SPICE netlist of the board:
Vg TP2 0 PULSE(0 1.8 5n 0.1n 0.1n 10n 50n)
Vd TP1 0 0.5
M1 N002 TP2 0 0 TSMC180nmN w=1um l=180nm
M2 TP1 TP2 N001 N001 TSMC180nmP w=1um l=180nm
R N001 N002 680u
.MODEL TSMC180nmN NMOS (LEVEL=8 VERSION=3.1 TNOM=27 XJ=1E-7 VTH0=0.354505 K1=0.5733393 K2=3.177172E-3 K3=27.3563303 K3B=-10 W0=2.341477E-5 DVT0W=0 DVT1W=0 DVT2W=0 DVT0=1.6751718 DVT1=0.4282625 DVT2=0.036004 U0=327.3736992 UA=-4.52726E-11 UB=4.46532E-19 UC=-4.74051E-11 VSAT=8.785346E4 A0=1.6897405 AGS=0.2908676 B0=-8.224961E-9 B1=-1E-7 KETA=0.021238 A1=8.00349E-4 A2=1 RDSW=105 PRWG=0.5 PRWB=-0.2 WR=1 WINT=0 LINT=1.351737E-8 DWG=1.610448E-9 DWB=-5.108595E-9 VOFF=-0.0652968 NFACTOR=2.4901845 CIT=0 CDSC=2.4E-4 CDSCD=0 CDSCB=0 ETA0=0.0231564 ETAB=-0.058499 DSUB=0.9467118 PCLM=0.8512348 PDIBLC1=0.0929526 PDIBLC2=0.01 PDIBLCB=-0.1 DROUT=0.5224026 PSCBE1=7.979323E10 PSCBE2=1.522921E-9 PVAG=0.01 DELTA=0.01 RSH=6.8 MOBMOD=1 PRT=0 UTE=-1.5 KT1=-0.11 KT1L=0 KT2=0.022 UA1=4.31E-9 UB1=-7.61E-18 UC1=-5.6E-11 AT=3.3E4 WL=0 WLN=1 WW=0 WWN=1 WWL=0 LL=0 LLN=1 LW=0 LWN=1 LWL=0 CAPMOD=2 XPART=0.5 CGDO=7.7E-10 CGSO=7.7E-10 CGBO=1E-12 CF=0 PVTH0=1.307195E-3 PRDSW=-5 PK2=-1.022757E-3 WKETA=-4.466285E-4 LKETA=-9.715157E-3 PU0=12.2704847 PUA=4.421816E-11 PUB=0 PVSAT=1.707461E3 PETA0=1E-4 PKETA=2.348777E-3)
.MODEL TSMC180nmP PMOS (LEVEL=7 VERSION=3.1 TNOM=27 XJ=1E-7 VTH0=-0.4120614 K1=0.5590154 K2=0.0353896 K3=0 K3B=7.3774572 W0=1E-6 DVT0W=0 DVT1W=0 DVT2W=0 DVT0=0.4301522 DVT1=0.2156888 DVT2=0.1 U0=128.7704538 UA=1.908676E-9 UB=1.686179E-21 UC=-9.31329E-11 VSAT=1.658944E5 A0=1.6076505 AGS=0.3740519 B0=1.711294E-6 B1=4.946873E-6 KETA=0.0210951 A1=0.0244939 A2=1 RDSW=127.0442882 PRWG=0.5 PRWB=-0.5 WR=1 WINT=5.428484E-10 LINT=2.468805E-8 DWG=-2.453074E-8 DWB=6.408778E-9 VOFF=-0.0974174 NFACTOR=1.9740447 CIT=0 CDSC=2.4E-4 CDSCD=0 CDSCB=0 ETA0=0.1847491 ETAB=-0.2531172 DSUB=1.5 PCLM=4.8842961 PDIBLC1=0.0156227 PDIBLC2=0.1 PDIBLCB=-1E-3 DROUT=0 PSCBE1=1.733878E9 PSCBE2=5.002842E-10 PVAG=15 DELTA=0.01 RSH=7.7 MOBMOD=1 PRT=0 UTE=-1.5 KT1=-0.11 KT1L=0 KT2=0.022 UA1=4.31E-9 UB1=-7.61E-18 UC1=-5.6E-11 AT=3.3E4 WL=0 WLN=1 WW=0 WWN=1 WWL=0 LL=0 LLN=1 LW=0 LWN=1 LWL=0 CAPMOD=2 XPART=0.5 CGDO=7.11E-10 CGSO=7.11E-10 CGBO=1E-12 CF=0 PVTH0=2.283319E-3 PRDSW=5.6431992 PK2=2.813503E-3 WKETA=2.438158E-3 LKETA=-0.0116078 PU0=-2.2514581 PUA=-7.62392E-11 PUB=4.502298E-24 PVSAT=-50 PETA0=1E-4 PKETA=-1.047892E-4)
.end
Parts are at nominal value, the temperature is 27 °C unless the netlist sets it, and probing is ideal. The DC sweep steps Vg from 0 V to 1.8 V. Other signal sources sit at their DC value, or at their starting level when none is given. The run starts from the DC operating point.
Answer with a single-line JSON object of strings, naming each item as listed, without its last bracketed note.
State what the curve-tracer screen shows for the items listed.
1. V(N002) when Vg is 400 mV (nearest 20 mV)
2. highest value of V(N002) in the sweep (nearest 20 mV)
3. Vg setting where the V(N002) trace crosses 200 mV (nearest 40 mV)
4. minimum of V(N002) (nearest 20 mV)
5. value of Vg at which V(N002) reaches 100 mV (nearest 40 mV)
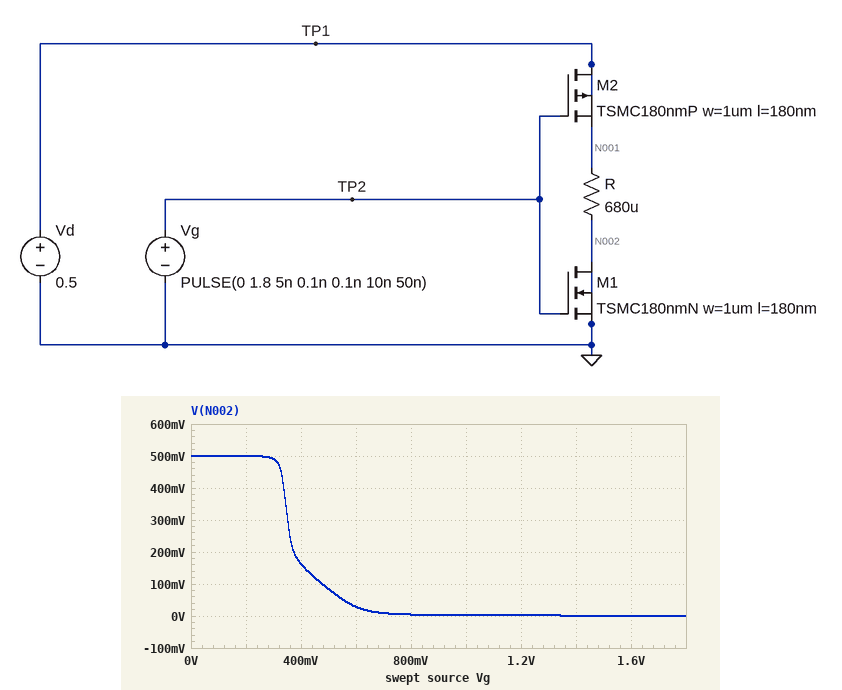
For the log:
{"V(N002) when Vg is 400 mV": "160 mV", "highest value of V(N002) in the sweep": "500 mV", "Vg setting where the V(N002) trace crosses 200 mV": "360 mV", "minimum of V(N002)": "0 V", "value of Vg at which V(N002) reaches 100 mV": "480 mV"}
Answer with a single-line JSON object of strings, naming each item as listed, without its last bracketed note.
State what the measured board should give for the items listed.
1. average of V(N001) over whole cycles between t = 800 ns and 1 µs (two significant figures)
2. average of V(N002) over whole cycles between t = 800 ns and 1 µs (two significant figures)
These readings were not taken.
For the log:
{"average of V(N001) over whole cycles between t = 800 ns and 1 µs": "390 mV", "average of V(N002) over whole cycles between t = 800 ns and 1 µs": "390 mV"}
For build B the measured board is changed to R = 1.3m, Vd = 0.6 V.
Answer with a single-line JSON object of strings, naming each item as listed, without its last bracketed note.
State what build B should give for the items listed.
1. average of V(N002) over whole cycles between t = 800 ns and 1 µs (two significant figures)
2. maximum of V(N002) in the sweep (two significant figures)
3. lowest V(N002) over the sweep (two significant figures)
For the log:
{"average of V(N002) over whole cycles between t = 800 ns and 1 µs": "480 mV", "maximum of V(N002) in the sweep": "600 mV", "lowest V(N002) over the sweep": "23 mV"}
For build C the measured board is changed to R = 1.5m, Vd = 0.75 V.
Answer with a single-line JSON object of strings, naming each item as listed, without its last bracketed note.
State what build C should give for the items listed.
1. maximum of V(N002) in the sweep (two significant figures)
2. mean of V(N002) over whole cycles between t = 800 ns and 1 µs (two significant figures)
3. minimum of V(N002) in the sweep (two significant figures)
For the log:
{"maximum of V(N002) in the sweep": "750 mV", "mean of V(N002) over whole cycles between t = 800 ns and 1 µs": "620 mV", "minimum of V(N002) in the sweep": "130 mV"}
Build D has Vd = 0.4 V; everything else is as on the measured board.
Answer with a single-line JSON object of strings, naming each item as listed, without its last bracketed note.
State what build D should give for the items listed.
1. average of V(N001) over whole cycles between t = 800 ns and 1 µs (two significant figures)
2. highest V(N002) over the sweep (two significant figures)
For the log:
{"average of V(N001) over whole cycles between t = 800 ns and 1 µs": "270 mV", "highest V(N002) over the sweep": "400 mV"}
